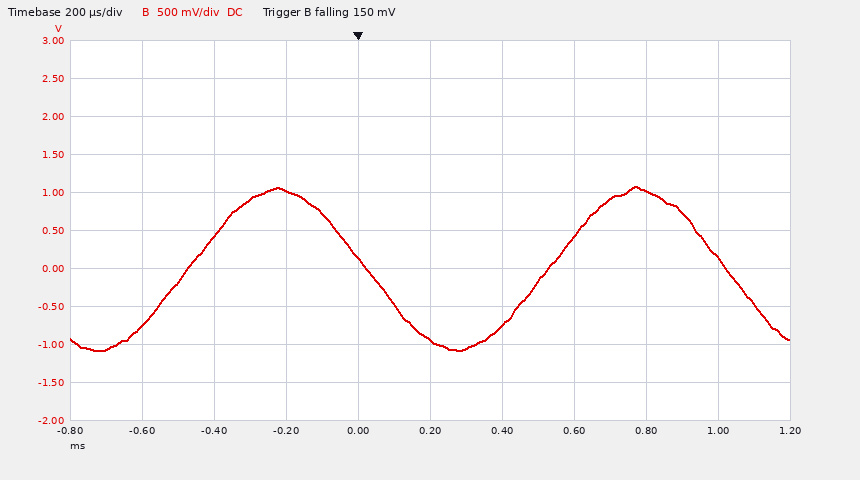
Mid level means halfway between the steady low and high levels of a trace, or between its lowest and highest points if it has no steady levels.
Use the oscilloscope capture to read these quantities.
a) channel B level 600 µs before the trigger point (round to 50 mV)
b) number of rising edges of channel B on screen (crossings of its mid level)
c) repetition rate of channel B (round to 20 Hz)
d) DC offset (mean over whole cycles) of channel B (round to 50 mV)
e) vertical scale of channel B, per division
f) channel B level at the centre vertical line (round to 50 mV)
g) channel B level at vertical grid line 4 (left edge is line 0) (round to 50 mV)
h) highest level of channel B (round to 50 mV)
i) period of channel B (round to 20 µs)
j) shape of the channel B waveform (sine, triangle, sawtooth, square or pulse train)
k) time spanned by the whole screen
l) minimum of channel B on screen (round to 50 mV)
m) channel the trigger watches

-750 mV
2
1.00 kHz
0 mV
500 mV
-950 mV
150 mV
1.10 V
1.00 ms
sine
2 ms
-1.10 V
channel B
